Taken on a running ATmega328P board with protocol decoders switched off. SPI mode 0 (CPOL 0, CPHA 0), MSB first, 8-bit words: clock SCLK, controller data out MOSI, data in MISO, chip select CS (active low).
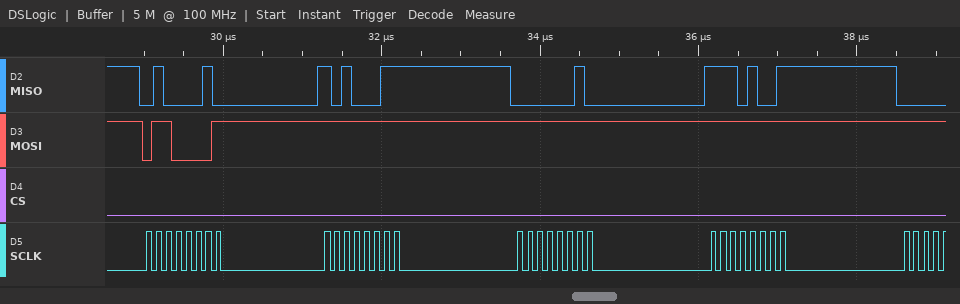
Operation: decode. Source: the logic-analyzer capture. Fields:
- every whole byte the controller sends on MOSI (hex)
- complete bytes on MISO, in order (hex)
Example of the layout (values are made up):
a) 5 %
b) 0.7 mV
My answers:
a) 61 FF FF FF
b) 42 A3 02 E9
